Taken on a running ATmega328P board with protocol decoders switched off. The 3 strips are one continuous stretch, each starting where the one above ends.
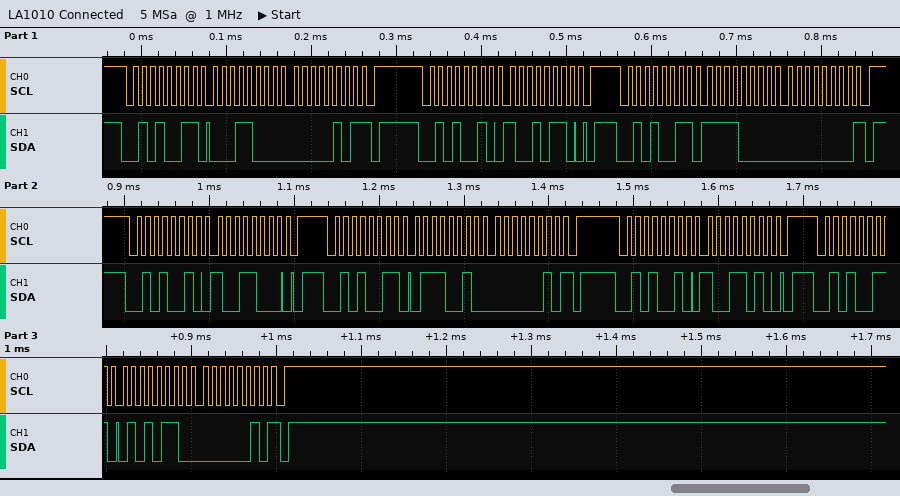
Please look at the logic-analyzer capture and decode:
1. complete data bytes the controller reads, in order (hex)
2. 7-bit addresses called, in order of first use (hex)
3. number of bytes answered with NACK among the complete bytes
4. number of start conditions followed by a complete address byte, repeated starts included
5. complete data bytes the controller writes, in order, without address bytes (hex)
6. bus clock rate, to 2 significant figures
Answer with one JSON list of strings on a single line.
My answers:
["18 05 F0 00 72 02 56 02", "0x29", "4", "7", "96 98 9A", "100 kHz"]
